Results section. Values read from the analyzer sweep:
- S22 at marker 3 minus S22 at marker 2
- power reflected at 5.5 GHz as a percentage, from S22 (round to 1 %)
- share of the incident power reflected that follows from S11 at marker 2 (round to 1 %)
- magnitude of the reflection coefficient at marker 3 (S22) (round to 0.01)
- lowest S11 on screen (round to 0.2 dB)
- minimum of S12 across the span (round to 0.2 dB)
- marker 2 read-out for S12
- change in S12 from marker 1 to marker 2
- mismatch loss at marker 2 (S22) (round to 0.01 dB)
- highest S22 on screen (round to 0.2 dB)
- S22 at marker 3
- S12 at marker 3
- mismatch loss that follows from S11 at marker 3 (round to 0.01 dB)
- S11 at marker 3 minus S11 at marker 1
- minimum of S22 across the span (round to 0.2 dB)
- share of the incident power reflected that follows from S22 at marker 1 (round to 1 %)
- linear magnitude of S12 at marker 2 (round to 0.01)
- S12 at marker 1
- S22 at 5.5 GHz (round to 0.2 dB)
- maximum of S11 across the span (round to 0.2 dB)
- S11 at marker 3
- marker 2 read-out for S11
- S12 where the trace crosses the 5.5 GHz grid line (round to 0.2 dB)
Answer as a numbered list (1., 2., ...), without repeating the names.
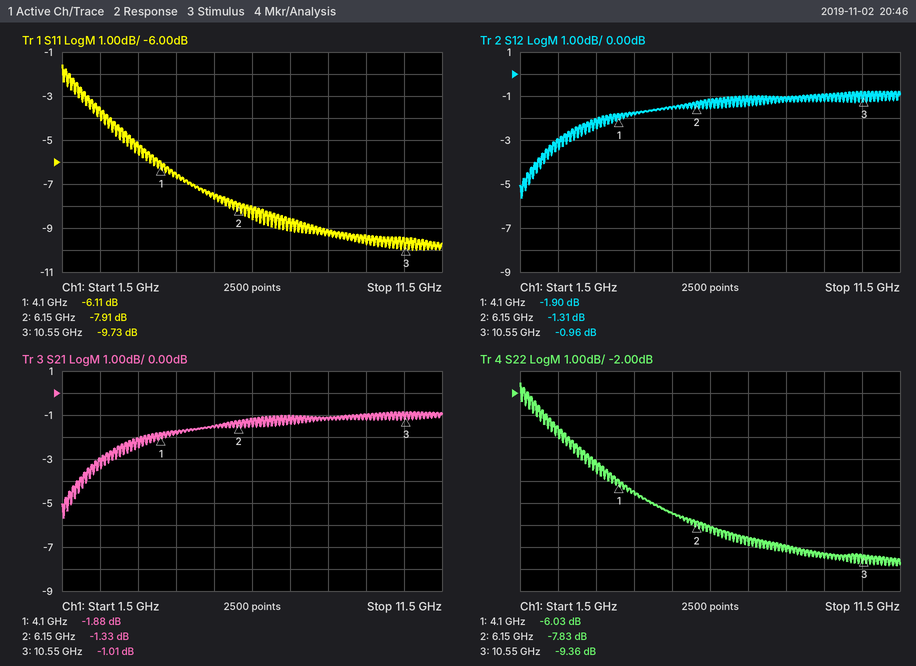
1. -1.53 dB
2. 18 %
3. 16 %
4. 0.34
5. -10.0 dB
6. -5.6 dB
7. -1.31 dB
8. 0.59 dB
9. 0.78 dB
10. -1.6 dB
11. -9.36 dB
12. -0.96 dB
13. 0.49 dB
14. -3.62 dB
15. -9.8 dB
16. 25 %
17. 0.86
18. -1.90 dB
19. -7.4 dB
20. -1.6 dB
21. -9.73 dB
22. -7.91 dB
23. -1.6 dB
